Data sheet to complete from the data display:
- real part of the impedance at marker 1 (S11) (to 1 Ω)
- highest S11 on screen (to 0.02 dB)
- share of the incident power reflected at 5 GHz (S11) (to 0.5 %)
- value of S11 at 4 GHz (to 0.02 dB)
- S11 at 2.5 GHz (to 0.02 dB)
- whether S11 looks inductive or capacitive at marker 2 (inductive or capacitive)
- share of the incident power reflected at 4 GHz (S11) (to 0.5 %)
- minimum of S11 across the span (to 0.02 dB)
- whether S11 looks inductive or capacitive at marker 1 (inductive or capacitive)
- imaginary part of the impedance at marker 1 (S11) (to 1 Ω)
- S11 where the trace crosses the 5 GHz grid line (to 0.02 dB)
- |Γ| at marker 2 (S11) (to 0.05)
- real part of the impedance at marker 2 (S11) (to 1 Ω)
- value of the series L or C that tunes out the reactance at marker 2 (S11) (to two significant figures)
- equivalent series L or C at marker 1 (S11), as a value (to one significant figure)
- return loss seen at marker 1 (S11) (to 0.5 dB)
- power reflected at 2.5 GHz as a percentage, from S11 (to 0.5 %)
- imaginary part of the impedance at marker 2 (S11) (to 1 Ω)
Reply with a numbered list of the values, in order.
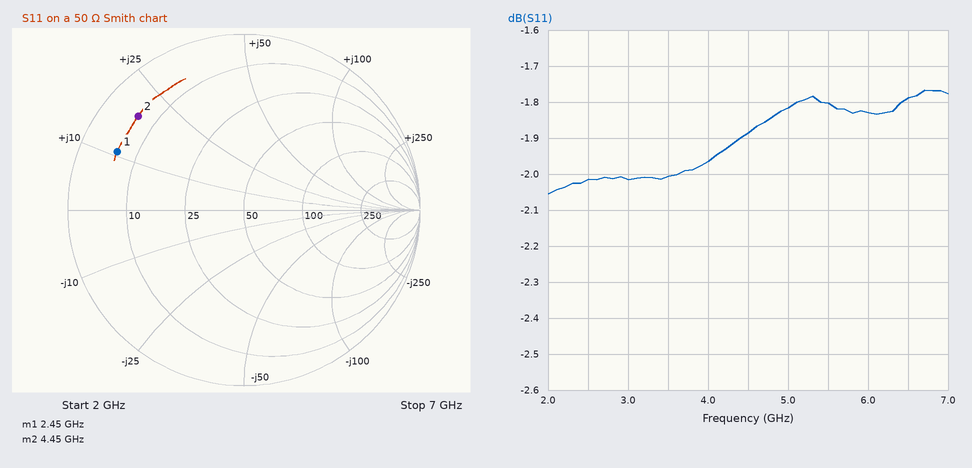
1. 6 Ω
2. -1.76 dB
3. 66.0 %
4. -1.96 dB
5. -2.02 dB
6. inductive
7. 63.5 %
8. -2.06 dB
9. inductive
10. +11 Ω
11. -1.82 dB
12. 0.80
13. 6 Ω
14. 1.9 pF
15. 700 pH
16. 2.0 dB
17. 63.0 %
18. +19 Ω
